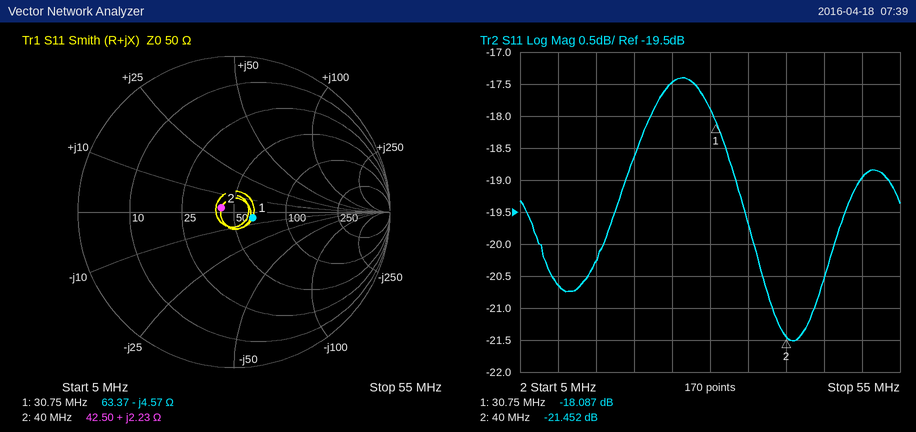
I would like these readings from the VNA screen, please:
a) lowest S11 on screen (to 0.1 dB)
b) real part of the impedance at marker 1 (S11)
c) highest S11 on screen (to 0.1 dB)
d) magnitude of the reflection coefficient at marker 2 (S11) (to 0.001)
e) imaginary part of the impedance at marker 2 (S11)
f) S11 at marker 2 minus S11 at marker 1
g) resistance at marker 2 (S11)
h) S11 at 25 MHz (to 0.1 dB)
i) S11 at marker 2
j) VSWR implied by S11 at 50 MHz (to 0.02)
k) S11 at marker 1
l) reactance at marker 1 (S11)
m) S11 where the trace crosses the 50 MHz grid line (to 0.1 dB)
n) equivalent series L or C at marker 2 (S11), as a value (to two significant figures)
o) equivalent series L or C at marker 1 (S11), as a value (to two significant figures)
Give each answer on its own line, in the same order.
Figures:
-21.5 dB
63.37 Ω
-17.4 dB
0.085
+2.23 Ω
-3.365 dB
42.50 Ω
-17.5 dB
-21.452 dB
1.26
-18.087 dB
-4.57 Ω
-19.0 dB
8.9 nH
1.1 nF
